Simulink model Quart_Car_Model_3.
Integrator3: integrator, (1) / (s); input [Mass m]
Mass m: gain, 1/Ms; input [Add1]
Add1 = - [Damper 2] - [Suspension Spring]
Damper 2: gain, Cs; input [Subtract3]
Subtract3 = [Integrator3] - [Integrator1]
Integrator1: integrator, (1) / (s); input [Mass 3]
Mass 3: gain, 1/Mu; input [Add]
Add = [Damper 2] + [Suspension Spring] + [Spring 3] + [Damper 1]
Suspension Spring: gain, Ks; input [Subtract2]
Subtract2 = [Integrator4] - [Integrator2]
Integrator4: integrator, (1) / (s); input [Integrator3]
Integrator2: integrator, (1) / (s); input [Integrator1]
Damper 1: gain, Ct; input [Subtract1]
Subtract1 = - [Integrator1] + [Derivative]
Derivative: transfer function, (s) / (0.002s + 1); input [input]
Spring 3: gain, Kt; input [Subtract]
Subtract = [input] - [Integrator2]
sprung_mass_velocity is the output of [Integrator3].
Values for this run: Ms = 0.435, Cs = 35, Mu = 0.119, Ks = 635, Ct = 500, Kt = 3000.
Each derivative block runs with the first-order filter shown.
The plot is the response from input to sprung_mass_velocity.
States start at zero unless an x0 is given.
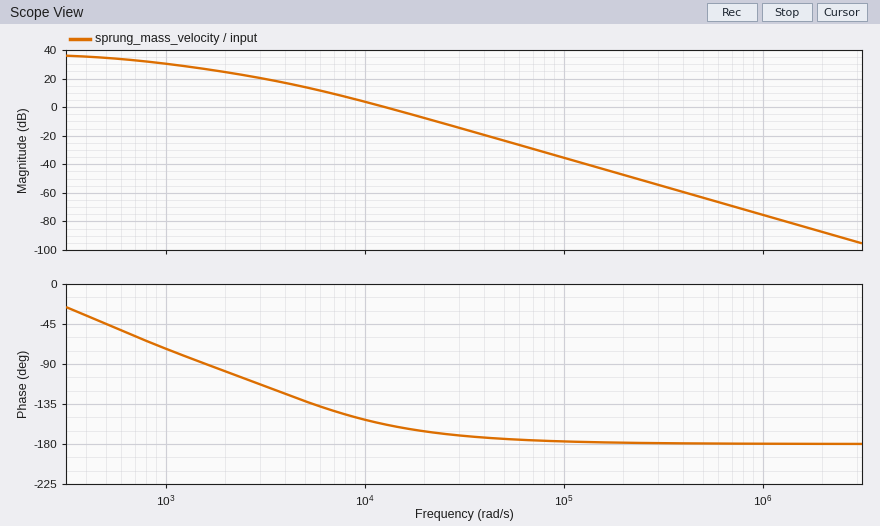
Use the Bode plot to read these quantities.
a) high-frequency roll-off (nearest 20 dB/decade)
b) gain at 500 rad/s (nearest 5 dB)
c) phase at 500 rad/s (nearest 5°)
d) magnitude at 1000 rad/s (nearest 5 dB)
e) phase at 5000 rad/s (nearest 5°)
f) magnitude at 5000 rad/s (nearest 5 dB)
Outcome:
-40 dB/decade
35 dB
-45°
30 dB
-130°
15 dB
